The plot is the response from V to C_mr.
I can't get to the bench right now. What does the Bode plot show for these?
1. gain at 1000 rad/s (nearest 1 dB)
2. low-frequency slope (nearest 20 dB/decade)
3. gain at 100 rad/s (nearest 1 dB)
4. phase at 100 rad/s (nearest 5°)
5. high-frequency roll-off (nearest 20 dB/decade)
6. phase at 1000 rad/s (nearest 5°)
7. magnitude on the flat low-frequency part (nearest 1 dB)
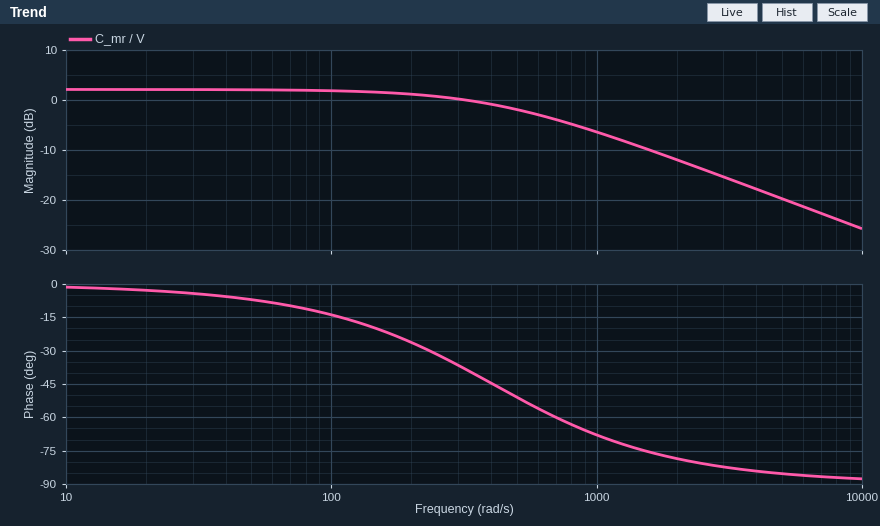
-6 dB
0 dB/decade
2 dB
-15°
-20 dB/decade
-70°
2 dB
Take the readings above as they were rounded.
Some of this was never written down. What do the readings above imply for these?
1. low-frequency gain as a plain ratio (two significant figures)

1.3
